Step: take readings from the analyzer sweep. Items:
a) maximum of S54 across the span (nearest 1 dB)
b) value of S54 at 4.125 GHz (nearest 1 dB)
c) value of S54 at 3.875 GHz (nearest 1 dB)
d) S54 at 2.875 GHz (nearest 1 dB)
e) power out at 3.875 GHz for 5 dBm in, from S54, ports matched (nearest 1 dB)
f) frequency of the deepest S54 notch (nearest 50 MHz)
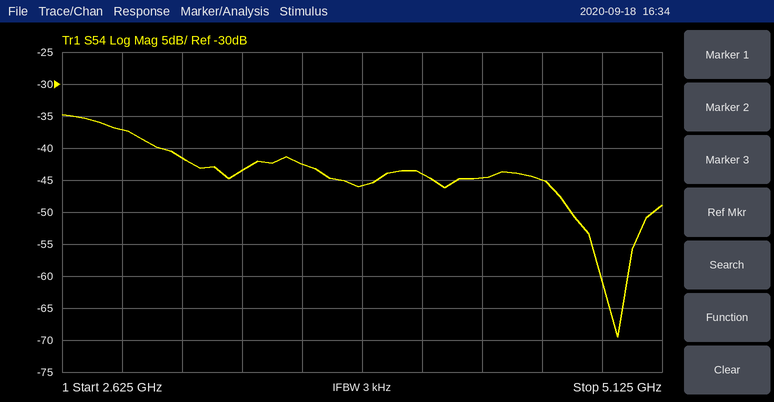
-35 dB
-44 dB
-46 dB
-37 dB
-41 dBm
4.95 GHz
